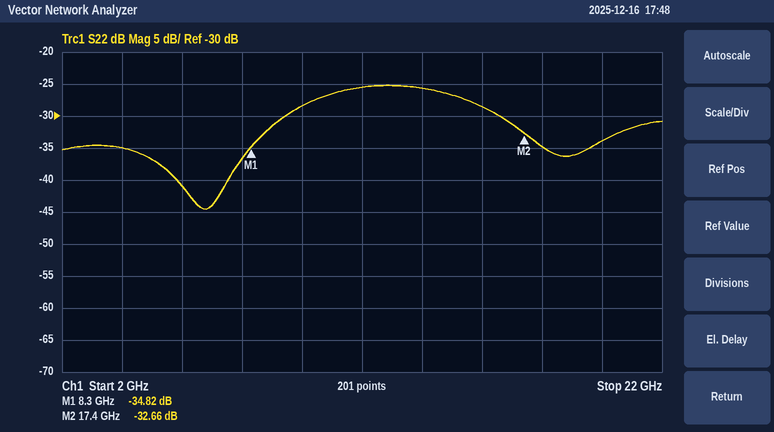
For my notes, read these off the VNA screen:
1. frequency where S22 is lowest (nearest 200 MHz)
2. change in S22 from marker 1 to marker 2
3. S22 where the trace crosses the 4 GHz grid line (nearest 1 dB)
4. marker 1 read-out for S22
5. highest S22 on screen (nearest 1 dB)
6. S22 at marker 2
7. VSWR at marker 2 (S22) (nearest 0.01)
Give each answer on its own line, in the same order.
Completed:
6.8 GHz
2.16 dB
-35 dB
-34.82 dB
-25 dB
-32.66 dB
1.05
